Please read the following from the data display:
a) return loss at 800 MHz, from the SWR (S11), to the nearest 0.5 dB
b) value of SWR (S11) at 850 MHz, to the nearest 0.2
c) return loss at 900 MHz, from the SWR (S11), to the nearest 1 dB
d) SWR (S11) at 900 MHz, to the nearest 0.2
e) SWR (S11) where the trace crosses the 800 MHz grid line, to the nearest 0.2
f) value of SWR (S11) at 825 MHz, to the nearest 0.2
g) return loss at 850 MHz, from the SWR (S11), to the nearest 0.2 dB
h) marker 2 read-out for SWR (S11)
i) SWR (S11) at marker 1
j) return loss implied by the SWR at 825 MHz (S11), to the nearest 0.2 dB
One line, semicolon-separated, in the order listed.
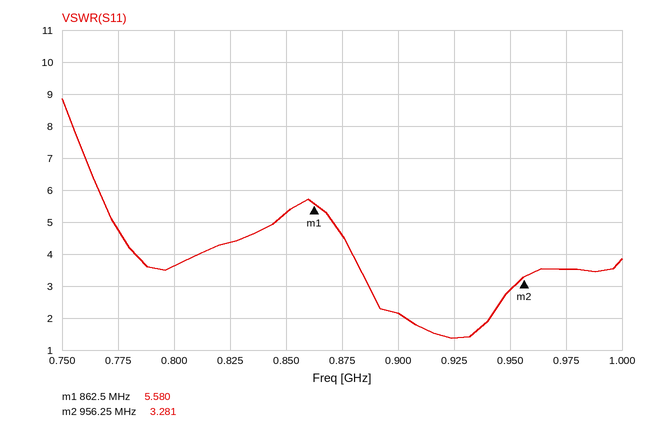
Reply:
5.0 dB; 5.2; 9 dB; 2.2; 3.6; 4.4; 3.4 dB; 3.281; 5.580; 4.0 dB
